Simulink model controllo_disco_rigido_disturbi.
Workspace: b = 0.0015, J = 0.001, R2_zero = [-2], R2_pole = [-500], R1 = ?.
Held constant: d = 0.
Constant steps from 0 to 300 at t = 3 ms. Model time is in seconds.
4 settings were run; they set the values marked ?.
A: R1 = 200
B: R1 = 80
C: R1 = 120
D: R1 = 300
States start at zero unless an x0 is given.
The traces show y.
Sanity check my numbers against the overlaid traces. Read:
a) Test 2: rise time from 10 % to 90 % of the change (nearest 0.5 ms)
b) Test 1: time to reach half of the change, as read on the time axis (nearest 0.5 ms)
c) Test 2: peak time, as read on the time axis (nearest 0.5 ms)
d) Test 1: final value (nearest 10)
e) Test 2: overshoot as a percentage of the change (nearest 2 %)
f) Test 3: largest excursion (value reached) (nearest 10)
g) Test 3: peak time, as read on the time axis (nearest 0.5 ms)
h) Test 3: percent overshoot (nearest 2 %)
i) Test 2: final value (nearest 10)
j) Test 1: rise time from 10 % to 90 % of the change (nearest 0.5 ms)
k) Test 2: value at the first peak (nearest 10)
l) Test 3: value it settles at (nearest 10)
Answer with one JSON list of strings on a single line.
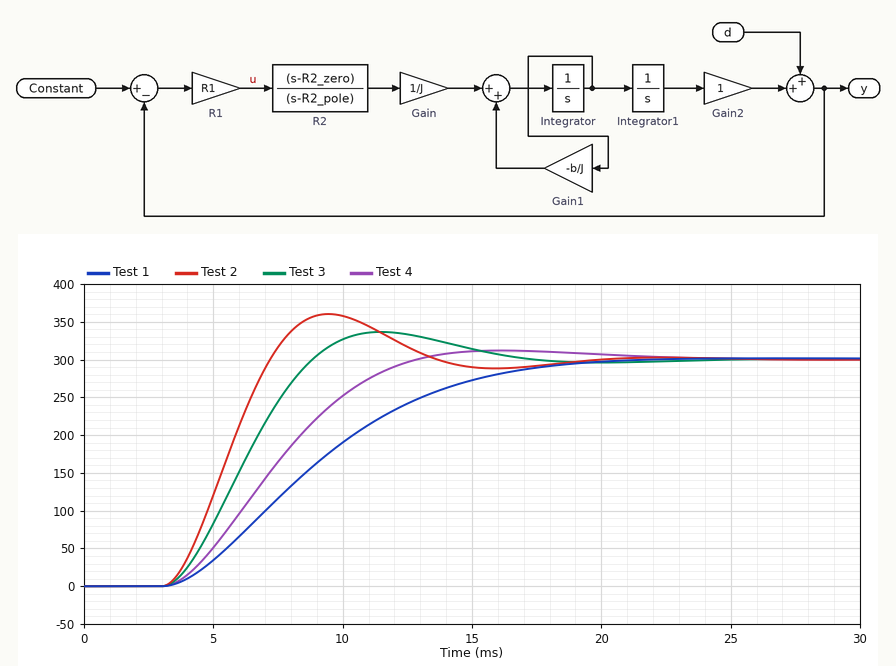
["3.0 ms", "8.5 ms", "9.5 ms", "300", "20 %", "340", "11.5 ms", "12 %", "300", "10.0 ms", "360", "300"]
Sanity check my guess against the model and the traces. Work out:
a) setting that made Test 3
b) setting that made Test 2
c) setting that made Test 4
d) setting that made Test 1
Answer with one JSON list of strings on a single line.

["A", "D", "C", "B"]
